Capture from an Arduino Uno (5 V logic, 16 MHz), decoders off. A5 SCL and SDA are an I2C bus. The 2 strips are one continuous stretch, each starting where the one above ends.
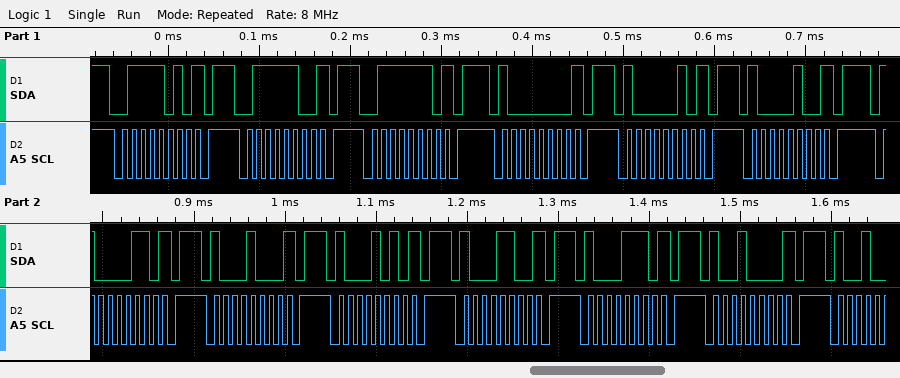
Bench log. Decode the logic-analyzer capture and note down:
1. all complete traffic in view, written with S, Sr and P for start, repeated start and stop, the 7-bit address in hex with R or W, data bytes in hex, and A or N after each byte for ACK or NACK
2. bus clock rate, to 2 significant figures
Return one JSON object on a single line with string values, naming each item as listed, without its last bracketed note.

{"all complete traffic in view, written with S, Sr and P for start, repeated start and stop, the 7-bit address in hex with R or W, data bytes in hex, and A or N after each byte for ACK or NACK": "S 3DW N P S 3EW N P S 3FW N P S 40W N P S 41W N P S 42W N P S 43W N P S 44W N P S 45W N P S 46W N P S 47W N P S 48W N P", "bus clock rate, to 2 significant figures": "100 kHz"}
